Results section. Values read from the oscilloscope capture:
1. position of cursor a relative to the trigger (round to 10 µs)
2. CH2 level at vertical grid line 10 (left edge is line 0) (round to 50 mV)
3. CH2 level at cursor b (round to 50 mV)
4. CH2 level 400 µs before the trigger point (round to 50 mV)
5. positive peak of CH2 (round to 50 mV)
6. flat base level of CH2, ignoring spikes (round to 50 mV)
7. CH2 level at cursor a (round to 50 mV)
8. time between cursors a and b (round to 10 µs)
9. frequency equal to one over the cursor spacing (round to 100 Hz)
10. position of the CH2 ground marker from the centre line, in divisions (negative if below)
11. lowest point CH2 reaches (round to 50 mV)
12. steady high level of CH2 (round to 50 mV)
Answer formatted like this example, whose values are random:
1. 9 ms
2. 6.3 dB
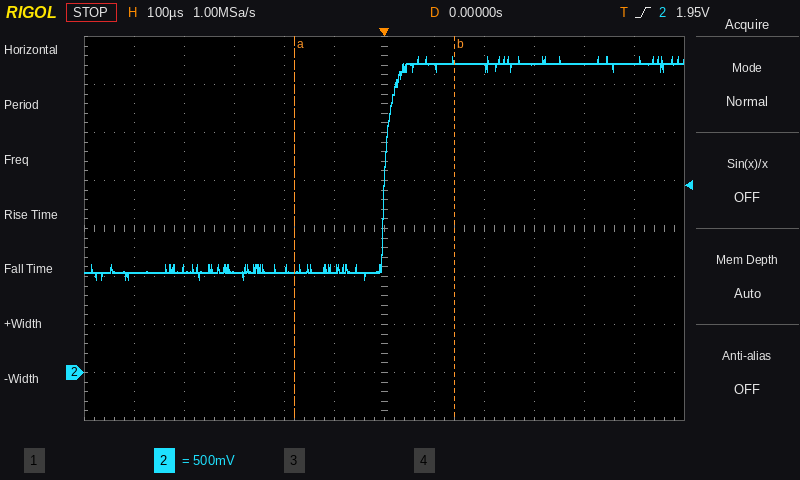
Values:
1. -180 µs
2. 3.20 V
3. 3.25 V
4. 1.10 V
5. 3.30 V
6. 1.05 V
7. 1.05 V
8. 320 µs
9. 3.1 kHz
10. -3.0 div
11. 950 mV
12. 3.20 V
